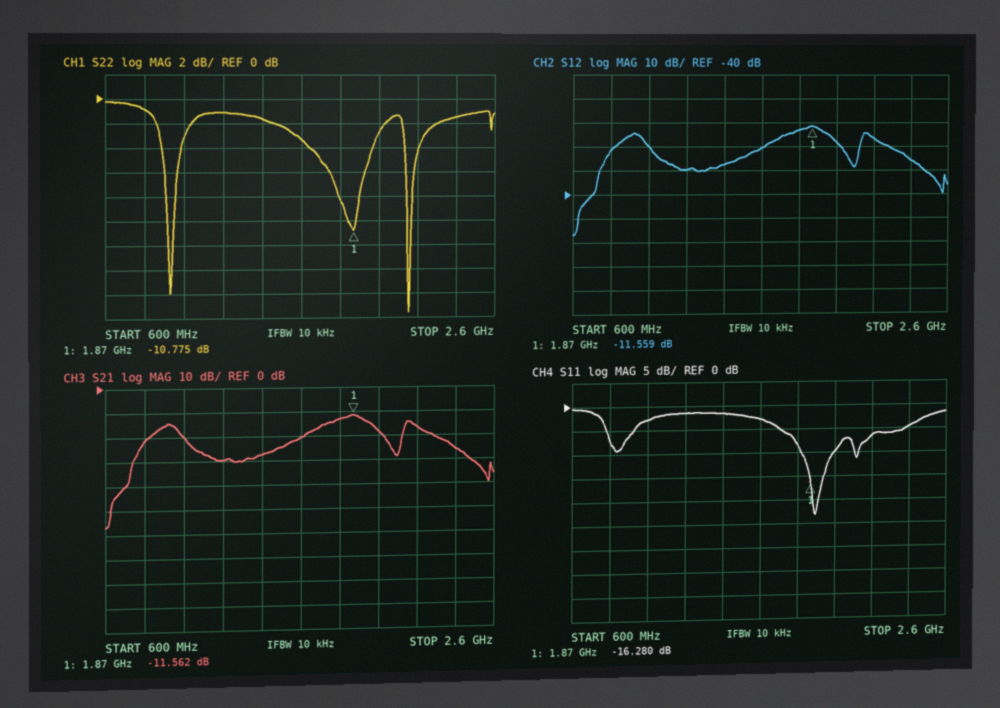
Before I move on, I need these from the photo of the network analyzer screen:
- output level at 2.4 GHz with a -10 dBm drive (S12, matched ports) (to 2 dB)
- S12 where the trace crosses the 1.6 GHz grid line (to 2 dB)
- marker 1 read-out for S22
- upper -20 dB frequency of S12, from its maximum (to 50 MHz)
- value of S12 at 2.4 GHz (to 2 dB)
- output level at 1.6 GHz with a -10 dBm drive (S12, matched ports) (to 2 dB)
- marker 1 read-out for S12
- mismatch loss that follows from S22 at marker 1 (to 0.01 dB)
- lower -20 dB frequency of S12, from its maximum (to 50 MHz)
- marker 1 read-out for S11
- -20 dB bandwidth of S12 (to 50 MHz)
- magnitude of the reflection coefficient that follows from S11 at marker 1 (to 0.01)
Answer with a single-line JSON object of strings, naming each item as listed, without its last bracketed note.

{"output level at 2.4 GHz with a -10 dBm drive (S12, matched ports)": "-36 dBm", "S12 where the trace crosses the 1.6 GHz grid line": "-20 dB", "marker 1 read-out for S22": "-10.775 dB", "upper -20 dB frequency of S12, from its maximum": "2.50 GHz", "value of S12 at 2.4 GHz": "-26 dB", "output level at 1.6 GHz with a -10 dBm drive (S12, matched ports)": "-30 dBm", "marker 1 read-out for S12": "-11.559 dB", "mismatch loss that follows from S22 at marker 1": "0.38 dB", "lower -20 dB frequency of S12, from its maximum": "750 MHz", "marker 1 read-out for S11": "-16.280 dB", "-20 dB bandwidth of S12": "1.75 GHz", "magnitude of the reflection coefficient that follows from S11 at marker 1": "0.15"}
